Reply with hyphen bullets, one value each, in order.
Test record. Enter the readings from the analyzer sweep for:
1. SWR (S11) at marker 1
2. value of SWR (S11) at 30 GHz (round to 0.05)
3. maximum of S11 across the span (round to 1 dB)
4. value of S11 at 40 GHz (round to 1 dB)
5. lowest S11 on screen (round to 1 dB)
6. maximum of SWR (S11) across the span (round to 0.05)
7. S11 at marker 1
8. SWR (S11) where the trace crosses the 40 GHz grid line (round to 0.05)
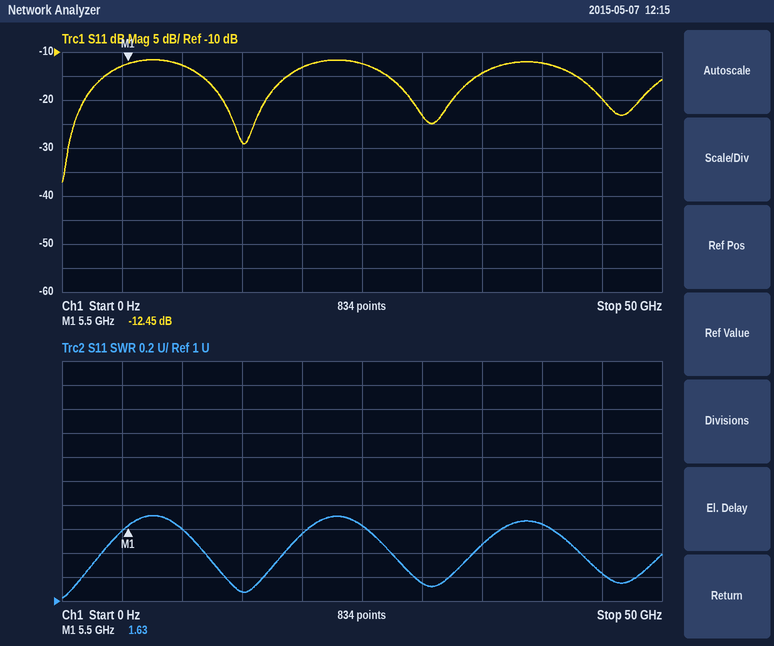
- 1.63
- 1.15
- -12 dB
- -12 dB
- -37 dB
- 1.70
- -12.45 dB
- 1.65
